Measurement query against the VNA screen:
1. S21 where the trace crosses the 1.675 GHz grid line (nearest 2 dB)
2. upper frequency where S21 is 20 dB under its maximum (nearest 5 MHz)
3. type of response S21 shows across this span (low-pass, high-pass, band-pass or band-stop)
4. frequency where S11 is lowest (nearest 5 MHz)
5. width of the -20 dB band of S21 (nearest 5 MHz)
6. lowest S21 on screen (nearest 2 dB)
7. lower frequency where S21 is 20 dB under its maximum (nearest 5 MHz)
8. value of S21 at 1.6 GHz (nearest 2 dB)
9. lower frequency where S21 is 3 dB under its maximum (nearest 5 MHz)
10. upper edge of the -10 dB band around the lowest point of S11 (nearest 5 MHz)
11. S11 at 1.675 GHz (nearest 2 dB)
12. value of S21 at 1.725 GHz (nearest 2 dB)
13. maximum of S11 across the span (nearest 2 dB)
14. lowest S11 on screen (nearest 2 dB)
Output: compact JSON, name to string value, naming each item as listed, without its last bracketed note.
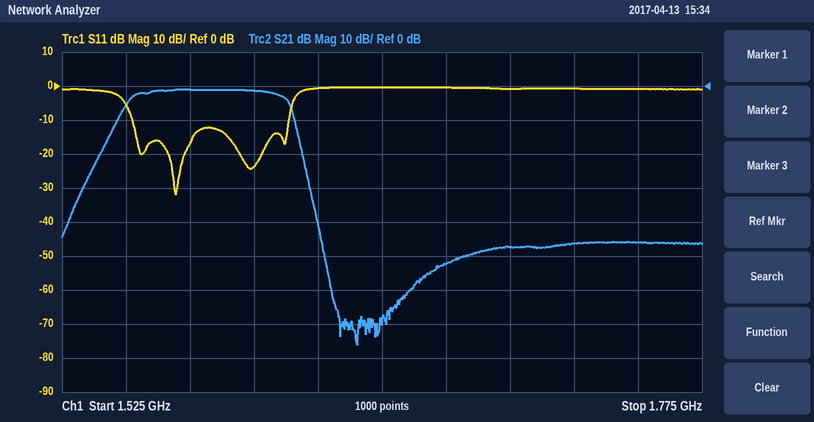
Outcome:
{"S21 where the trace crosses the 1.675 GHz grid line": "-52 dB", "upper frequency where S21 is 20 dB under its maximum": "1.620 GHz", "type of response S21 shows across this span": "band-pass", "frequency where S11 is lowest": "1.570 GHz", "width of the -20 dB band of S21": "80 MHz", "lowest S21 on screen": "-76 dB", "lower frequency where S21 is 20 dB under its maximum": "1.540 GHz", "value of S21 at 1.6 GHz": "-2 dB", "lower frequency where S21 is 3 dB under its maximum": "1.550 GHz", "upper edge of the -10 dB band around the lowest point of S11": "1.615 GHz", "S11 at 1.675 GHz": "0 dB", "value of S21 at 1.725 GHz": "-46 dB", "maximum of S11 across the span": "0 dB", "lowest S11 on screen": "-32 dB"}
